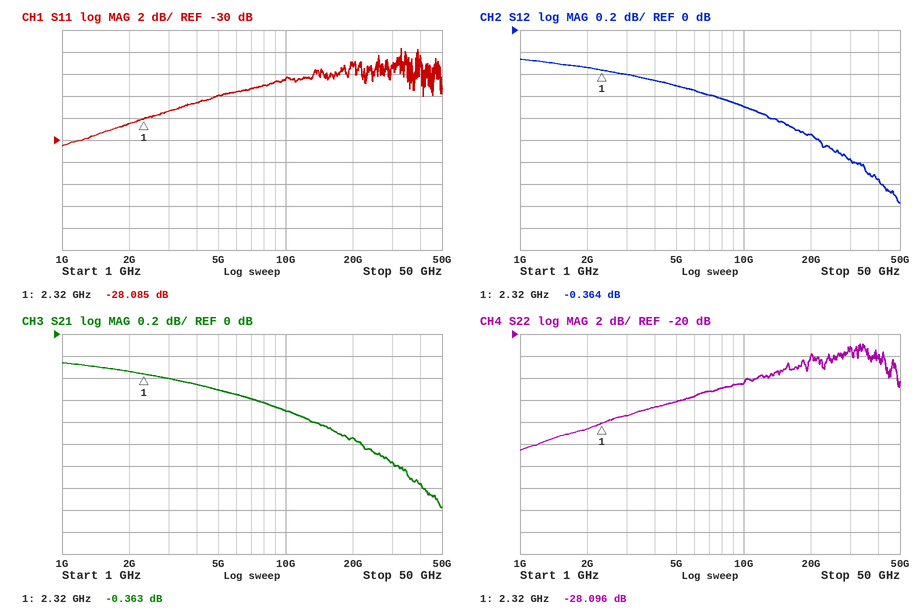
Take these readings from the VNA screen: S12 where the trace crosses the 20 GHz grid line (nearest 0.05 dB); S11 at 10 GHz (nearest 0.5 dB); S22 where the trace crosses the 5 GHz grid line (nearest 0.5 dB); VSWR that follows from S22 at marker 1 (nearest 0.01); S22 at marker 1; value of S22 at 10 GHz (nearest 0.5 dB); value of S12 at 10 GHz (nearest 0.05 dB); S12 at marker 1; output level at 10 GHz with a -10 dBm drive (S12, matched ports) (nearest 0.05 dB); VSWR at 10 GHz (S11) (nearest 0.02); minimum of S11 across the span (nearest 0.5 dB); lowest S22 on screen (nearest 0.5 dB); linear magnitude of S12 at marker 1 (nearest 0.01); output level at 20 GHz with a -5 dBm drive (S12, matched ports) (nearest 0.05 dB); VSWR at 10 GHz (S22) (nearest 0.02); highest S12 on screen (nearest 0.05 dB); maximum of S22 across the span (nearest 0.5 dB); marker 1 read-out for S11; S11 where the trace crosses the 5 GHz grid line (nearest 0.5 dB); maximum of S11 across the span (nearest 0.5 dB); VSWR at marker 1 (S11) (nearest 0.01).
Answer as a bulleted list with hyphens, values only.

- -0.95 dB
- -24.5 dB
- -26.0 dB
- 1.08
- -28.096 dB
- -24.5 dB
- -0.70 dB
- -0.364 dB
- -10.70 dBm
- 1.12
- -30.5 dB
- -30.5 dB
- 0.96
- -5.95 dBm
- 1.12
- -0.25 dB
- -21.0 dB
- -28.085 dB
- -26.0 dB
- -21.5 dB
- 1.08
